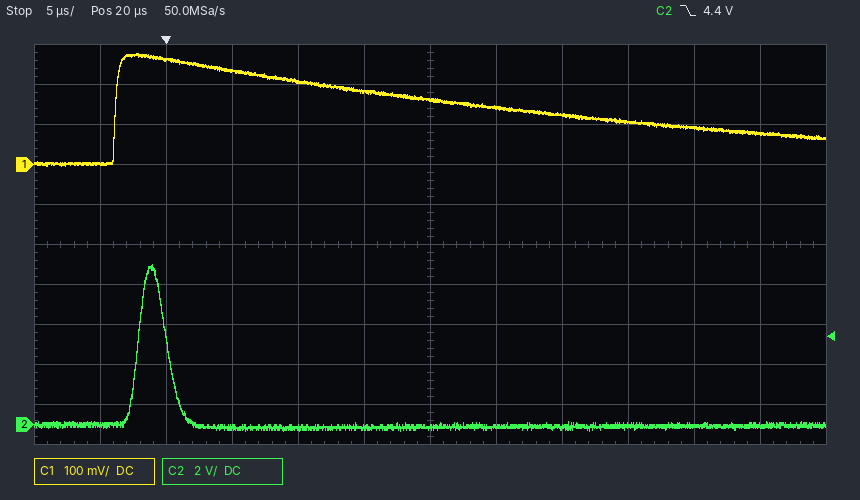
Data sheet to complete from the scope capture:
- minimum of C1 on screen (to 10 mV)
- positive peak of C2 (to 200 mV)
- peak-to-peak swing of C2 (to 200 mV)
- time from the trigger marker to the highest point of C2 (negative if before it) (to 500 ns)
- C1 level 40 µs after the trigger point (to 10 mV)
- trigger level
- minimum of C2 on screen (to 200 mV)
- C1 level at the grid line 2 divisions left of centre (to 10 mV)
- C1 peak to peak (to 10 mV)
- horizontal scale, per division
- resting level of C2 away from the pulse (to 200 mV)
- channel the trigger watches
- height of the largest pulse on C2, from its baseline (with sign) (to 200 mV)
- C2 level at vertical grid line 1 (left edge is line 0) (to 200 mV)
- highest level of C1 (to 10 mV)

0 mV
8.0 V
8.4 V
-1.0 µs
90 mV
4.4 V
-400 mV
210 mV
280 mV
5 µs
0.0 V
C2
+8.0 V
0.0 V
280 mV
